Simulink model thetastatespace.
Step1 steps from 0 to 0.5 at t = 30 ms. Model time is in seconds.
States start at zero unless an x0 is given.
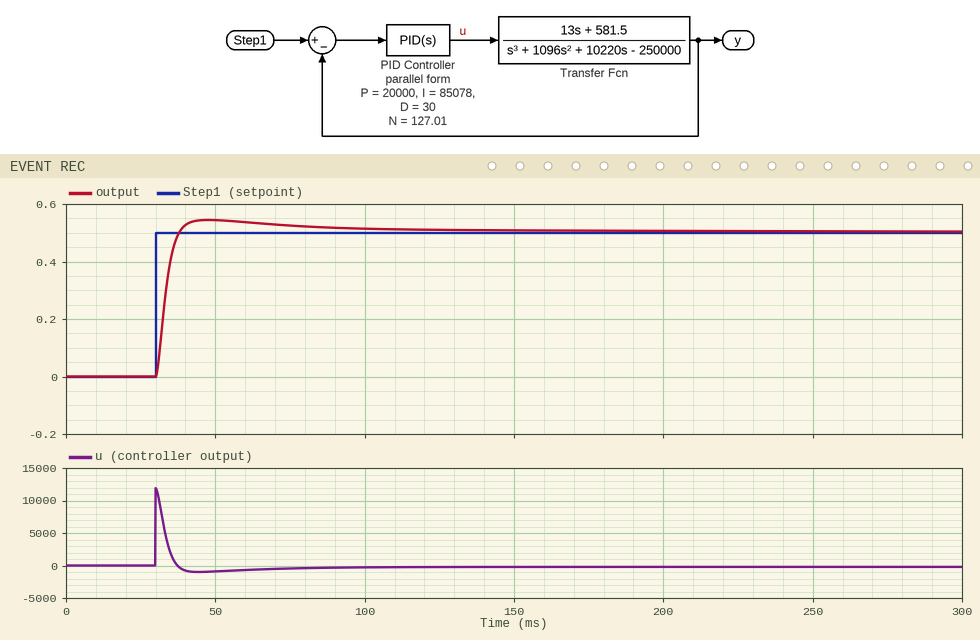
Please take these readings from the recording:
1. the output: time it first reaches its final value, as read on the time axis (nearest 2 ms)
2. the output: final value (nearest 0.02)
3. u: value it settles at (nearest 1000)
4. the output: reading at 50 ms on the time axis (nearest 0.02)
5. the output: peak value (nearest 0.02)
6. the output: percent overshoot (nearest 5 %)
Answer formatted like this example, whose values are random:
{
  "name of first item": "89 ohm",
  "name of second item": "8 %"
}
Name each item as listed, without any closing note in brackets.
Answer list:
{
  "the output: time it first reaches its final value, as read on the time axis": "38 ms",
  "the output: final value": "0.50",
  "u: value it settles at": "0",
  "the output: reading at 50 ms on the time axis": "0.54",
  "the output: peak value": "0.54",
  "the output: percent overshoot": "10 %"
}
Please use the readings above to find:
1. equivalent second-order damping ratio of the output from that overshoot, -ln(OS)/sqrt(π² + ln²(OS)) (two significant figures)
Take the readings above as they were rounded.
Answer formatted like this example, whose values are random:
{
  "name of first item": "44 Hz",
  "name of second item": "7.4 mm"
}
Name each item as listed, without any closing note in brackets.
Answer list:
{
  "equivalent second-order damping ratio of the output from that overshoot, -ln(OS)/sqrt(π² + ln²(OS))": "0.59"
}
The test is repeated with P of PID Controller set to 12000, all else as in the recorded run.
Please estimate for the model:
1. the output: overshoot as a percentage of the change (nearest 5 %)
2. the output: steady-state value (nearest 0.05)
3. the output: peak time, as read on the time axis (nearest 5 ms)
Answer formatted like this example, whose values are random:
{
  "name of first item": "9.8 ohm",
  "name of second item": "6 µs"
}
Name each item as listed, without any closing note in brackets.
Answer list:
{
  "the output: overshoot as a percentage of the change": "15 %",
  "the output: steady-state value": "0.50",
  "the output: peak time, as read on the time axis": "60 ms"
}
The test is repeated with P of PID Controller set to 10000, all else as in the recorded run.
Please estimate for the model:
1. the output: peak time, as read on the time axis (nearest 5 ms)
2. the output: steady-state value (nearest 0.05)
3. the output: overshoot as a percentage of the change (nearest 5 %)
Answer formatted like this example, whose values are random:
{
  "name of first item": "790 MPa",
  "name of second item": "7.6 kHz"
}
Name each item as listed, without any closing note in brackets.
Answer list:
{
  "the output: peak time, as read on the time axis": "60 ms",
  "the output: steady-state value": "0.50",
  "the output: overshoot as a percentage of the change": "15 %"
}
